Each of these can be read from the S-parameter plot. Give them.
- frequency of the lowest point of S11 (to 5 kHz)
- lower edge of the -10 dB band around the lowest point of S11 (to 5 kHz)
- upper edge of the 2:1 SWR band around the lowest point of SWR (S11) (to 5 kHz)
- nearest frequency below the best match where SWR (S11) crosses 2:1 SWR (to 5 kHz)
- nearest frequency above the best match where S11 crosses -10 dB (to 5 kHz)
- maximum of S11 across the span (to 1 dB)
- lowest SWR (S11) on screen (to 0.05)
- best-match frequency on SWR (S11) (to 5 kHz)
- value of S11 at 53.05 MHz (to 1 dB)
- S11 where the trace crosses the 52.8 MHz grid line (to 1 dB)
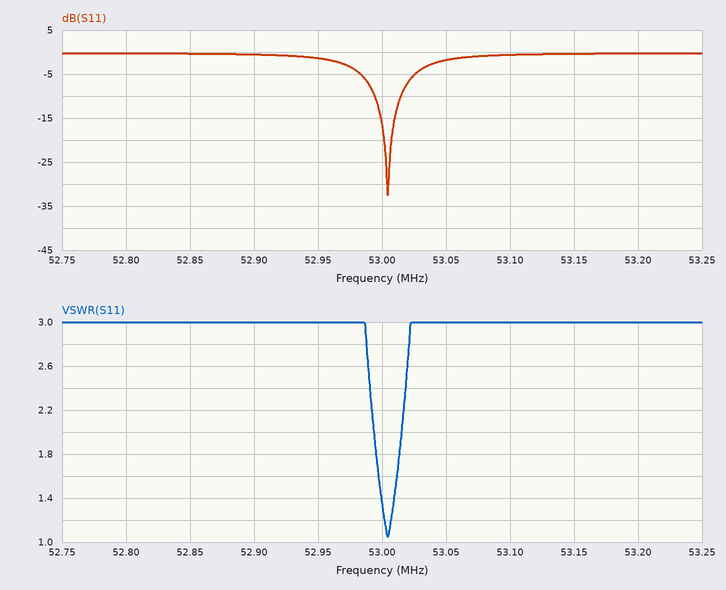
53.005 MHz
52.995 MHz
53.015 MHz
52.995 MHz
53.015 MHz
0 dB
1.05
53.005 MHz
-2 dB
0 dB
